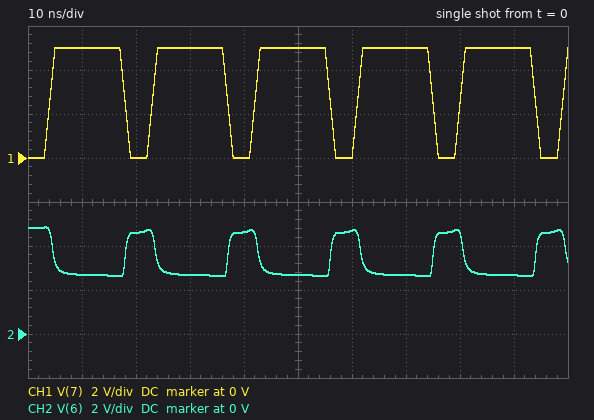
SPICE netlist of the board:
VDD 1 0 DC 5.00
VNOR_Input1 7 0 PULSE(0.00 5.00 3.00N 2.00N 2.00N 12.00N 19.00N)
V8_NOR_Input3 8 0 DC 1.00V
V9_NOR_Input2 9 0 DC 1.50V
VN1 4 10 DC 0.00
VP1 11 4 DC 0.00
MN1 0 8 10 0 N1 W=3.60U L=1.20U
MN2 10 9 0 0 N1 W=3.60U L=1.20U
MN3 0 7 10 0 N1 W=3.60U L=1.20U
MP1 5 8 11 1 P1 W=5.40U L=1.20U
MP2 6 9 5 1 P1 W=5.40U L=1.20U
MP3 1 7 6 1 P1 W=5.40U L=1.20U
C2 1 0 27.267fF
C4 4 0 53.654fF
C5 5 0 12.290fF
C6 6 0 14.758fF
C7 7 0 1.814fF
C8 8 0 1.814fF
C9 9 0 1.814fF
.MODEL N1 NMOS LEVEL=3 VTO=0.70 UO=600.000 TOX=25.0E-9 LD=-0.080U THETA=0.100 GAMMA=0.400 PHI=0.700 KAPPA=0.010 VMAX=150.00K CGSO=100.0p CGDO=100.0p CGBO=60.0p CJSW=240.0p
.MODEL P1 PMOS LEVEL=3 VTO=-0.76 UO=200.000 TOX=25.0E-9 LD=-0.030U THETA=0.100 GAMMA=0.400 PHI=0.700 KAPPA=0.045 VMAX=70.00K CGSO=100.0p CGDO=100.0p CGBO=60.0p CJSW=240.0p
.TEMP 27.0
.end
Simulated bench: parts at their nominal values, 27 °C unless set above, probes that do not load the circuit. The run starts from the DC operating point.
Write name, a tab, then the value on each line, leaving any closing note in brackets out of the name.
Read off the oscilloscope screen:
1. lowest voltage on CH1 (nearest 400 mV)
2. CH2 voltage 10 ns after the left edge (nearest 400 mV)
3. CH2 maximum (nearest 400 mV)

lowest voltage on CH1	0 V
CH2 voltage 10 ns after the left edge	2.8 V
CH2 maximum	4.8 V
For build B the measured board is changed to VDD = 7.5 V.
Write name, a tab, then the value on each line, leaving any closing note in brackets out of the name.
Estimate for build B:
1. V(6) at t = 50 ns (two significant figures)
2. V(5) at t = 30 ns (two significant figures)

V(6) at t = 50 ns	4.7 V
V(5) at t = 30 ns	3.9 V
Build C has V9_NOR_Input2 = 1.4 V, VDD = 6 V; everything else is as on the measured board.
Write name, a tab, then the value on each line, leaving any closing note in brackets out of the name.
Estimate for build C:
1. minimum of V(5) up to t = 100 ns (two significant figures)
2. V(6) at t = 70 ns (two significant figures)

minimum of V(5) up to t = 100 ns	2.5 V
V(6) at t = 70 ns	2.8 V
